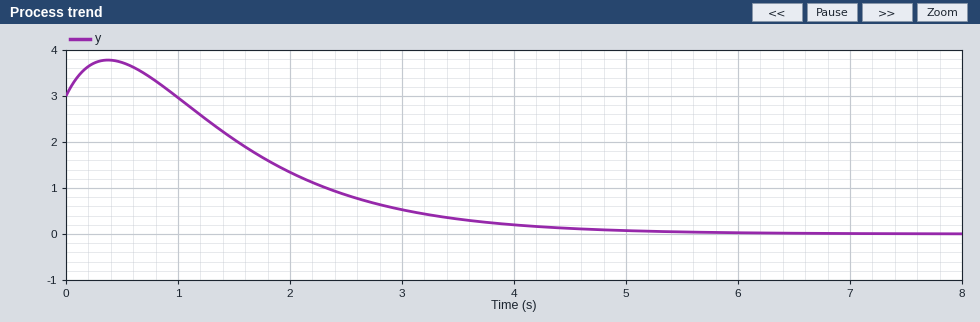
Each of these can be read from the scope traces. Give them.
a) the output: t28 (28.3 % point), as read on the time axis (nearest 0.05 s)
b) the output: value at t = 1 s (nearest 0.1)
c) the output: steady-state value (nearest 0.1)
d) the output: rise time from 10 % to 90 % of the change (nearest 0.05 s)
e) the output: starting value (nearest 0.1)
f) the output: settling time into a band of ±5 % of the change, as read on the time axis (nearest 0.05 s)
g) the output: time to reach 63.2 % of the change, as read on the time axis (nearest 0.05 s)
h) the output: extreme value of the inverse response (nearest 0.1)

1.45 s
3.0
0.0
2.45 s
3.0
4.30 s
2.20 s
3.8
